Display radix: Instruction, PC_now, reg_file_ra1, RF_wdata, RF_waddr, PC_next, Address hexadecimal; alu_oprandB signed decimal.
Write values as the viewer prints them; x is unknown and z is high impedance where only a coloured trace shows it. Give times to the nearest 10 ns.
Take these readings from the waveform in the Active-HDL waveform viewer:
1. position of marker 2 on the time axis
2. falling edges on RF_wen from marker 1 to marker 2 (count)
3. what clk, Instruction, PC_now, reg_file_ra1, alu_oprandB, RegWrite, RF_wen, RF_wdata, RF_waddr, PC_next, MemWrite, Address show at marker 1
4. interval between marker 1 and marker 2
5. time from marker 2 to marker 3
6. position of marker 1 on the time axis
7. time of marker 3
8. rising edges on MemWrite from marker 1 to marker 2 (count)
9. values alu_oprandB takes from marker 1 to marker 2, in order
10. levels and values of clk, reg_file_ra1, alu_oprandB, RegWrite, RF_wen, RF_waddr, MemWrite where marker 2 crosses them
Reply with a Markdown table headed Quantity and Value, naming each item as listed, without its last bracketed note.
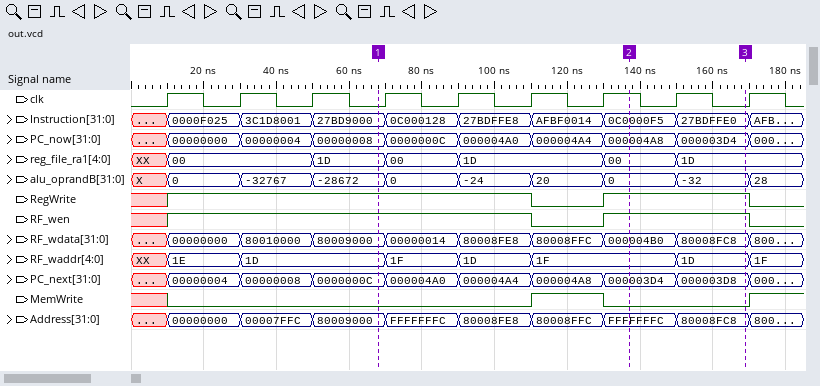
| Quantity | Value |
|---|---|
| position of marker 2 on the time axis | 140 ns |
| falling edges on RF_wen from marker 1 to marker 2 | 1 |
| what clk, Instruction, PC_now, reg_file_ra1, alu_oprandB, RegWrite, RF_wen, RF_wdata, RF_waddr, PC_next, MemWrite, Address show at marker 1 | clk=0, Instruction=27BD9000, PC_now=00000008, reg_file_ra1=1D, alu_oprandB=-28672, RegWrite=1, RF_wen=1, RF_wdata=80009000, RF_waddr=1D, PC_next=0000000C, MemWrite=0, Address=80009000 |
| interval between marker 1 and marker 2 | 70 ns |
| time from marker 2 to marker 3 | 30 ns |
| position of marker 1 on the time axis | 70 ns |
| time of marker 3 | 170 ns |
| rising edges on MemWrite from marker 1 to marker 2 | 1 |
| values alu_oprandB takes from marker 1 to marker 2, in order | -28672, 0, -24, 20, 0 |
| levels and values of clk, reg_file_ra1, alu_oprandB, RegWrite, RF_wen, RF_waddr, MemWrite where marker 2 crosses them | clk=1, reg_file_ra1=00, alu_oprandB=0, RegWrite=1, RF_wen=1, RF_waddr=1F, MemWrite=0 |
